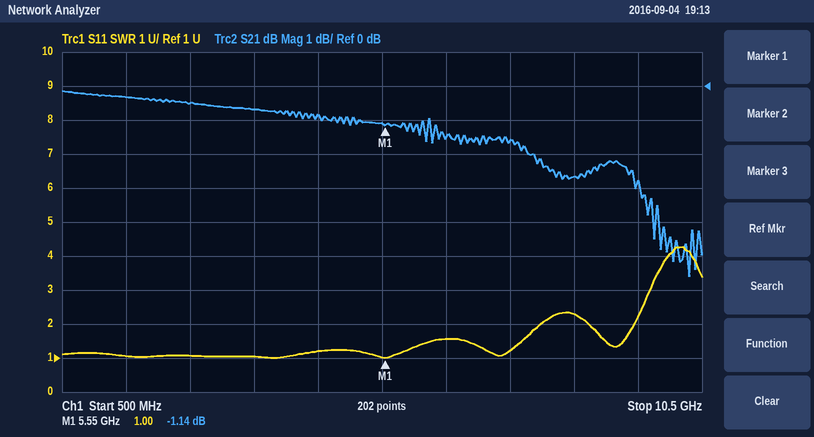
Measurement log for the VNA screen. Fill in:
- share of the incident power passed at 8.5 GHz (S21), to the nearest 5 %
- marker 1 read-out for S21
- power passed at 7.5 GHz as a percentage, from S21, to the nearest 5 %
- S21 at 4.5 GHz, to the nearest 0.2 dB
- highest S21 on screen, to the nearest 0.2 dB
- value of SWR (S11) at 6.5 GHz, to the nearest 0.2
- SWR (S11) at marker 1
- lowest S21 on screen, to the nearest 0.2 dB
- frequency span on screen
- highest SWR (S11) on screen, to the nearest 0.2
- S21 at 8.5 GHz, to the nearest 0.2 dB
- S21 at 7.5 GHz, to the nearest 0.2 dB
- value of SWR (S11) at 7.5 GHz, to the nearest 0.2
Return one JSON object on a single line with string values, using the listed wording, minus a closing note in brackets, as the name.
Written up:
{"share of the incident power passed at 8.5 GHz (S21), to the nearest 5 %": "55 %", "marker 1 read-out for S21": "-1.14 dB", "power passed at 7.5 GHz as a percentage, from S21, to the nearest 5 %": "70 %", "S21 at 4.5 GHz, to the nearest 0.2 dB": "-0.8 dB", "highest S21 on screen, to the nearest 0.2 dB": "-0.2 dB", "value of SWR (S11) at 6.5 GHz, to the nearest 0.2": "1.6", "SWR (S11) at marker 1": "1.00", "lowest S21 on screen, to the nearest 0.2 dB": "-5.6 dB", "frequency span on screen": "10 GHz", "highest SWR (S11) on screen, to the nearest 0.2": "4.2", "S21 at 8.5 GHz, to the nearest 0.2 dB": "-2.6 dB", "S21 at 7.5 GHz, to the nearest 0.2 dB": "-1.6 dB", "value of SWR (S11) at 7.5 GHz, to the nearest 0.2": "1.2"}
